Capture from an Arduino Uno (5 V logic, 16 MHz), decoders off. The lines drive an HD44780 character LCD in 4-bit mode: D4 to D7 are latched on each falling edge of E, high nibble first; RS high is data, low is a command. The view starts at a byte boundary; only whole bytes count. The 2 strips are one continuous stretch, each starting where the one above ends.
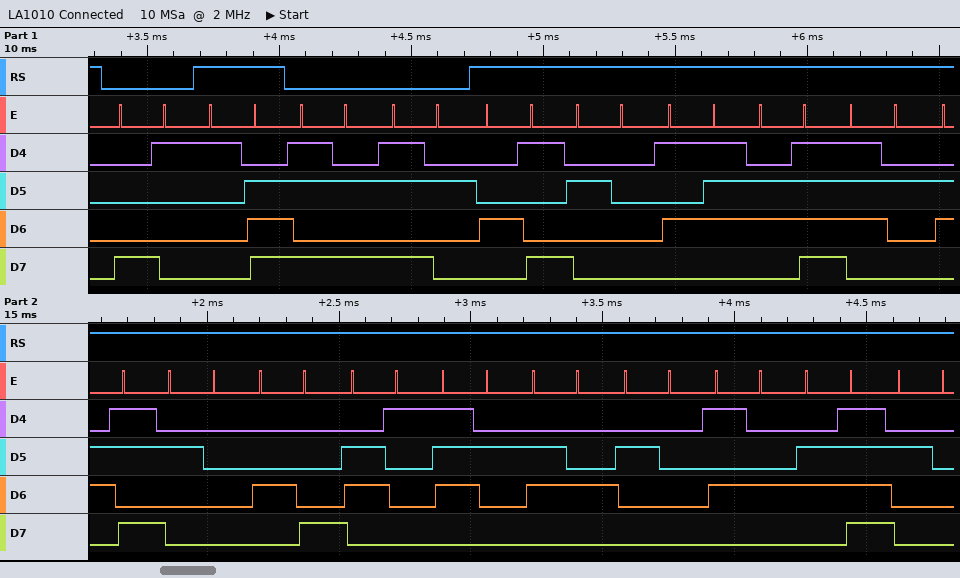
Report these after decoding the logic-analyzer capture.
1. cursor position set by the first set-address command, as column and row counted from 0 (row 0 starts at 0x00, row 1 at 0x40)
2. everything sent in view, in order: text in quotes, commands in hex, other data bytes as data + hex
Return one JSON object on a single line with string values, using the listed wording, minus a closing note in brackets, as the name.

{"cursor position set by the first set-address command, as column and row counted from 0": "column 1, row 0", "everything sent in view, in order: text in quotes, commands in hex, other data bytes as data + hex": "0x81 data 1E 0xBA 0xB2 \"I Work Hard To \""}
